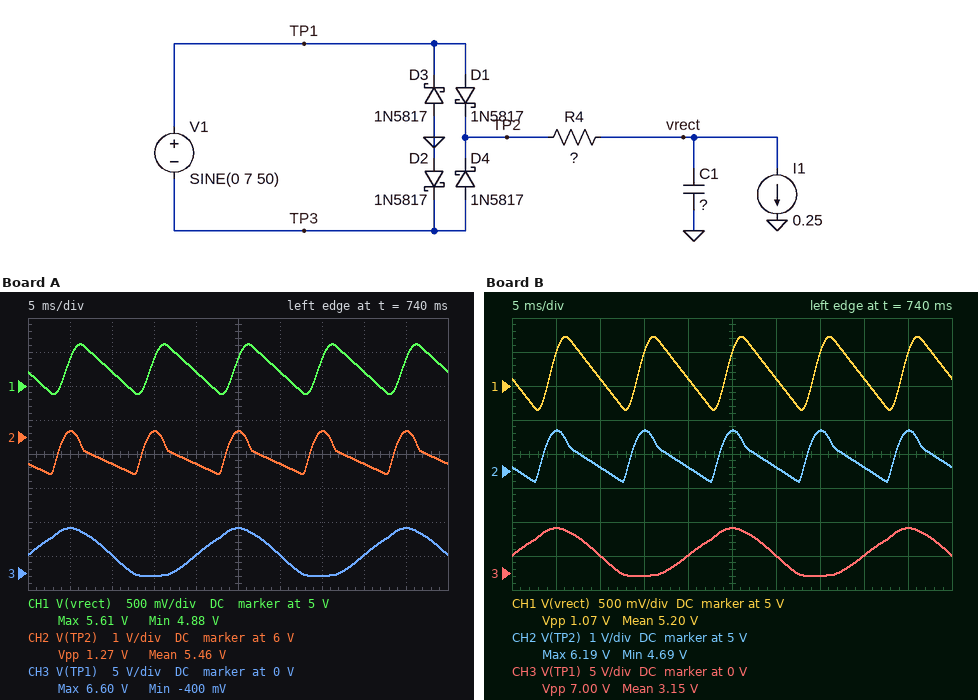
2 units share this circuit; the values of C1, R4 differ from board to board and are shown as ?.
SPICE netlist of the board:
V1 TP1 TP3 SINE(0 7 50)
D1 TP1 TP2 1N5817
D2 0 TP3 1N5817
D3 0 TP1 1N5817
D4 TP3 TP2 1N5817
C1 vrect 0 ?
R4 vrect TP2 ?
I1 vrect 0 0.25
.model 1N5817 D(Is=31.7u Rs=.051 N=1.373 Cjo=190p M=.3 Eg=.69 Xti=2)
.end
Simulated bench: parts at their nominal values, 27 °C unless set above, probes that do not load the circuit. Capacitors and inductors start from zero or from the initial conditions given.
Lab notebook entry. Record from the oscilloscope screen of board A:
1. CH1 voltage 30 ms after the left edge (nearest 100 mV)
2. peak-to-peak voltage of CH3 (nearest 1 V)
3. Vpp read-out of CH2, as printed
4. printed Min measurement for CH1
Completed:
5.2 V
7 V
1.27 V
4.88 V
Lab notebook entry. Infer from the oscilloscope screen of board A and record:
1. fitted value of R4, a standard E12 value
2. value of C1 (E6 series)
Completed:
0.82 Ω
2.2 mF
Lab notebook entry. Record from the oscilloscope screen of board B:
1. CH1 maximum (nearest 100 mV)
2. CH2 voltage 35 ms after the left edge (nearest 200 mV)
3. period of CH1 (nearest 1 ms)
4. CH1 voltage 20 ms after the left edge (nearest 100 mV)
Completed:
5.7 V
6.2 V
10 ms
5.1 V
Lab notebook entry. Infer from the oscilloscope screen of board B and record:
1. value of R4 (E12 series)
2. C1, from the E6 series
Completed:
0.82 Ω
1.5 mF
